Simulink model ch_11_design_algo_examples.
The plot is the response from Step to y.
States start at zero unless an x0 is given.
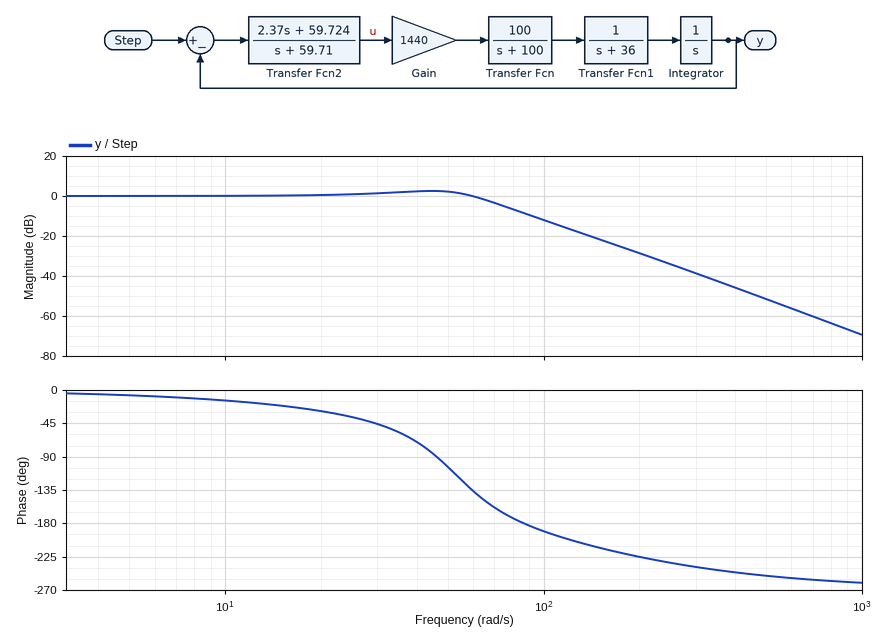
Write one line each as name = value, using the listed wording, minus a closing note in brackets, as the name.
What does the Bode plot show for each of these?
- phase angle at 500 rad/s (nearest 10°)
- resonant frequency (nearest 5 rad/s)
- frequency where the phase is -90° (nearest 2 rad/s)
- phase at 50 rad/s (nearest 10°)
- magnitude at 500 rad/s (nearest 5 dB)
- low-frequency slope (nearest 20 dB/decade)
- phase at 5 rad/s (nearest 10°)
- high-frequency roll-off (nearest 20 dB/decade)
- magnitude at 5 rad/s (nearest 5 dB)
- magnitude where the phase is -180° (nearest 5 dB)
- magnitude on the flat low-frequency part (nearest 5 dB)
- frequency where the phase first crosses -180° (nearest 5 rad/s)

phase angle at 500 rad/s = -250°
resonant frequency = 45 rad/s
frequency where the phase is -90° = 46 rad/s
phase at 50 rad/s = -100°
magnitude at 500 rad/s = -50 dB
low-frequency slope = 0 dB/decade
phase at 5 rad/s = -10°
high-frequency roll-off = -60 dB/decade
magnitude at 5 rad/s = 0 dB
magnitude where the phase is -180° = -10 dB
magnitude on the flat low-frequency part = 0 dB
frequency where the phase first crosses -180° = 85 rad/s
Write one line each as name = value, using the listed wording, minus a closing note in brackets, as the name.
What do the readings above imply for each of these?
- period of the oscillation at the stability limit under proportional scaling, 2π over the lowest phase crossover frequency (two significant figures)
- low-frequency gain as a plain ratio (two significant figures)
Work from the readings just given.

period of the oscillation at the stability limit under proportional scaling, 2π over the lowest phase crossover frequency = 0.074 s
low-frequency gain as a plain ratio = 1.0
